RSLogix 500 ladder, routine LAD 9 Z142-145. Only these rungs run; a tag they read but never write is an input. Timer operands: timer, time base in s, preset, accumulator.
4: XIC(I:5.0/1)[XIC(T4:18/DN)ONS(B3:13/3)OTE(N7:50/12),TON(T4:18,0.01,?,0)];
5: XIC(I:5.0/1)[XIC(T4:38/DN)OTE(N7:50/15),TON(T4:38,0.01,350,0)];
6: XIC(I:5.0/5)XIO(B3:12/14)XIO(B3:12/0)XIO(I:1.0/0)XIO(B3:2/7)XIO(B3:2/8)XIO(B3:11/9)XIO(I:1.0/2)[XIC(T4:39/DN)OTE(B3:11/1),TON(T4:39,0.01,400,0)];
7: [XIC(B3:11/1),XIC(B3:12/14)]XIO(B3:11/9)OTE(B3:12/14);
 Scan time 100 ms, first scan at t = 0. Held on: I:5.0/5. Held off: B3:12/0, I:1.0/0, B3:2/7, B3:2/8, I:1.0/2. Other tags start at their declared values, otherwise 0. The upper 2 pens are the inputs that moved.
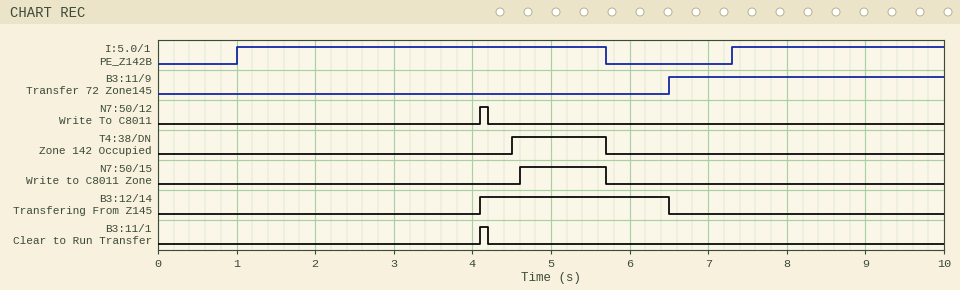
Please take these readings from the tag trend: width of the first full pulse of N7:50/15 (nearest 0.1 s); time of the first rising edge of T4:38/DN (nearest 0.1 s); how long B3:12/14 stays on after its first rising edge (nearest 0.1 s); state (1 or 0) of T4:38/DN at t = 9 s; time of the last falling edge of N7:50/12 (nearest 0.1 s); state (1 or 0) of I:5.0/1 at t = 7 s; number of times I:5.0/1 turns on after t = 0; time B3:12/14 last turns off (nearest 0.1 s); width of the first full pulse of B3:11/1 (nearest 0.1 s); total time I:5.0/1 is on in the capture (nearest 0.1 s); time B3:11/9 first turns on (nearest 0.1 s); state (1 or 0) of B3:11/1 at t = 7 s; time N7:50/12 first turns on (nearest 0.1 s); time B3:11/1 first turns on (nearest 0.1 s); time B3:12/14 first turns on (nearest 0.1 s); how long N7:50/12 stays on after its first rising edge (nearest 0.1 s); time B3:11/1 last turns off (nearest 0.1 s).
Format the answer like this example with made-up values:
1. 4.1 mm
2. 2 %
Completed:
1. 1.1 s
2. 4.5 s
3. 2.4 s
4. 0
5. 4.2 s
6. 0
7. 2
8. 6.5 s
9. 0.1 s
10. 7.4 s
11. 6.5 s
12. 0
13. 4.1 s
14. 4.1 s
15. 4.1 s
16. 0.1 s
17. 4.2 s
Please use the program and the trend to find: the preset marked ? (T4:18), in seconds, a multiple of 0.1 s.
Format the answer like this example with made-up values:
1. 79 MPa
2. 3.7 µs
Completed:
1. 3.0 s
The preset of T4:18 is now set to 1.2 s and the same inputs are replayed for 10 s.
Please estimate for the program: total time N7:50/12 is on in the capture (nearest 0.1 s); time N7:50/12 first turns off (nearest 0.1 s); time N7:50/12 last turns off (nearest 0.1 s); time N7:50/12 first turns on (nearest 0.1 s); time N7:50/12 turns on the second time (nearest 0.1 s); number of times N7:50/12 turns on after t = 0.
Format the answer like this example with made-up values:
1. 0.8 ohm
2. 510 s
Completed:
1. 0.2 s
2. 2.4 s
3. 8.7 s
4. 2.3 s
5. 8.6 s
6. 2
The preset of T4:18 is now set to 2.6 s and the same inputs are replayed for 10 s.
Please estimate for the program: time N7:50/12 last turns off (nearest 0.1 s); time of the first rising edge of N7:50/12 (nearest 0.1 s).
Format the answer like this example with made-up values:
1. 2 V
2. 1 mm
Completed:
1. 3.8 s
2. 3.7 s
